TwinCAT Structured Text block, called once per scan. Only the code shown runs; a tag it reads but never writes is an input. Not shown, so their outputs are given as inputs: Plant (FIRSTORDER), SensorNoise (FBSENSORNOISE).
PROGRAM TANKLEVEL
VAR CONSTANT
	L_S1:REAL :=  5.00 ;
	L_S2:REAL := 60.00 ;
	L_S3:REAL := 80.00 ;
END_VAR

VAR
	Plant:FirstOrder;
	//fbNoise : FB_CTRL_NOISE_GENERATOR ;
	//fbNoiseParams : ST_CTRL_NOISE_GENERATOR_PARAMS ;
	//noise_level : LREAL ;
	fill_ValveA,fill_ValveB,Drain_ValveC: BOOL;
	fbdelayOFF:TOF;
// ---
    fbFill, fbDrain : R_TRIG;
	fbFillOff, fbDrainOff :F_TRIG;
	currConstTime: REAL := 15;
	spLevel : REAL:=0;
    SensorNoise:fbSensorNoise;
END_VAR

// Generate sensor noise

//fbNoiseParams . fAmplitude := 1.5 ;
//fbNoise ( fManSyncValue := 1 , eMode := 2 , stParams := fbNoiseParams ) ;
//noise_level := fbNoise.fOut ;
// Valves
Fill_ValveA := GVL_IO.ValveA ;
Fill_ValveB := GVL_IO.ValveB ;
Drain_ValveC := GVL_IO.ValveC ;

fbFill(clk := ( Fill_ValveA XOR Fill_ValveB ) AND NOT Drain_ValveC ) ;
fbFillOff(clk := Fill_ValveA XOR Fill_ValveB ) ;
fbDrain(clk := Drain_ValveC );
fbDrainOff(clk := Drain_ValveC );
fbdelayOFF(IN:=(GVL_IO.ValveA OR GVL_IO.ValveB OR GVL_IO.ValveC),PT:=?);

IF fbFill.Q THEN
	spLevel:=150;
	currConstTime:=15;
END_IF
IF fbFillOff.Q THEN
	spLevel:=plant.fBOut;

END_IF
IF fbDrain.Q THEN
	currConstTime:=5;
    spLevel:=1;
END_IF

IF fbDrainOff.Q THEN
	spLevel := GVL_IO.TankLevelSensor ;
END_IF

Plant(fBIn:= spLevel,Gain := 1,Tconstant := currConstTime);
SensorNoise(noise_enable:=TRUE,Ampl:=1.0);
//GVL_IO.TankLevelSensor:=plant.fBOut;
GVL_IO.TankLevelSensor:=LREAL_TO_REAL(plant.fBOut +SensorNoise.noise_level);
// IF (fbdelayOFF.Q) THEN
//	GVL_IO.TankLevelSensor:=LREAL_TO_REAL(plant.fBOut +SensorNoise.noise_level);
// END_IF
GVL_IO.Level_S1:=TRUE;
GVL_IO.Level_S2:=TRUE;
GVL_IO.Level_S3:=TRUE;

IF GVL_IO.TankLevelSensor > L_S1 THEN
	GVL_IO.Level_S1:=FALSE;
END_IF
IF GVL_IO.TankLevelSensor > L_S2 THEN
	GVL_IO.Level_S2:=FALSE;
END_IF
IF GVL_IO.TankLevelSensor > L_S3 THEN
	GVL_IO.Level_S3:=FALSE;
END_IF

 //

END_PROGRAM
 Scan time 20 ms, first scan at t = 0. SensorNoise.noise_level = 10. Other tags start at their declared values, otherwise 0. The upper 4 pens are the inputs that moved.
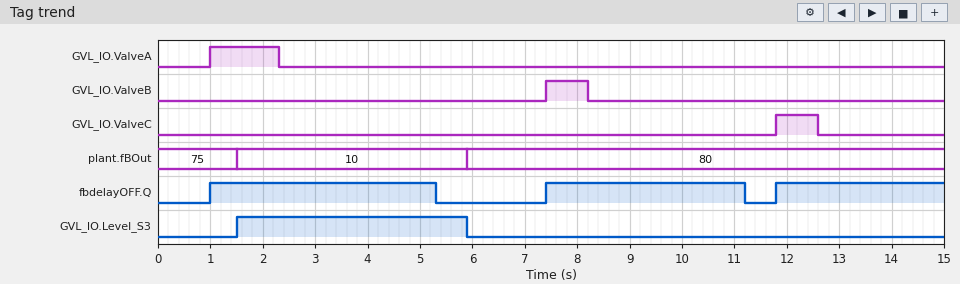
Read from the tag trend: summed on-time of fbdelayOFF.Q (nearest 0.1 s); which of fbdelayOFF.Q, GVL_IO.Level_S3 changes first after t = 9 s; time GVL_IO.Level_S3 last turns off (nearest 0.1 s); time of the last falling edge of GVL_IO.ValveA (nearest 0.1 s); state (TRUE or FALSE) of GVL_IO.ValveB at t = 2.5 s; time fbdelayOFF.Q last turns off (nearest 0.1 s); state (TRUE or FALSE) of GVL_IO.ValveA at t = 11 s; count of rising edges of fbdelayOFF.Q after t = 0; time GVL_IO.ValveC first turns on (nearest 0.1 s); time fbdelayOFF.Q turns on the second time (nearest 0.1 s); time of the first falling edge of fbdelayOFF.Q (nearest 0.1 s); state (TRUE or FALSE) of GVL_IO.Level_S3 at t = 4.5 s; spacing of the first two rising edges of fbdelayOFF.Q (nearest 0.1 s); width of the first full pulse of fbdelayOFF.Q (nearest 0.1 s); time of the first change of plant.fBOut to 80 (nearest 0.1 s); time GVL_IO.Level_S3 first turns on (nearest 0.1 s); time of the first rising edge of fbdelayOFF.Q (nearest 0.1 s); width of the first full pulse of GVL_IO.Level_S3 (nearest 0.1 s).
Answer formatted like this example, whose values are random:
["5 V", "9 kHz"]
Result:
["11.3 s", "fbdelayOFF.Q", "5.9 s", "2.3 s", "FALSE", "11.2 s", "FALSE", "3", "11.8 s", "7.4 s", "5.3 s", "TRUE", "6.4 s", "4.3 s", "5.9 s", "1.5 s", "1.0 s", "4.4 s"]
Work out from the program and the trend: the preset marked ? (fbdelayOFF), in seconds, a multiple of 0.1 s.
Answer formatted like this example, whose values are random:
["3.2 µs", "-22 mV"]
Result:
["3.0 s"]
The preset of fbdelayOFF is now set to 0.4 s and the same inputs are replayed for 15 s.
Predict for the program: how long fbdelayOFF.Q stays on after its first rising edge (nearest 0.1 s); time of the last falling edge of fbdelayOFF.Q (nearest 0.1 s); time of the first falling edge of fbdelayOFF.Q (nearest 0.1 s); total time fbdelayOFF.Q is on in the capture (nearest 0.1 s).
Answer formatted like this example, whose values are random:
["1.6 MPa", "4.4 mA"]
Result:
["1.7 s", "13.0 s", "2.7 s", "4.1 s"]
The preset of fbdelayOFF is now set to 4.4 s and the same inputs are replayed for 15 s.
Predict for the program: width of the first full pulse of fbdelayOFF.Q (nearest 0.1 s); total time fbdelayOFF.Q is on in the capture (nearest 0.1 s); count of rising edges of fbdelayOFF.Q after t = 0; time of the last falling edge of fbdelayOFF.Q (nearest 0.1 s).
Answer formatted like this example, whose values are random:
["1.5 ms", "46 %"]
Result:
["5.7 s", "13.3 s", "2", "6.7 s"]
